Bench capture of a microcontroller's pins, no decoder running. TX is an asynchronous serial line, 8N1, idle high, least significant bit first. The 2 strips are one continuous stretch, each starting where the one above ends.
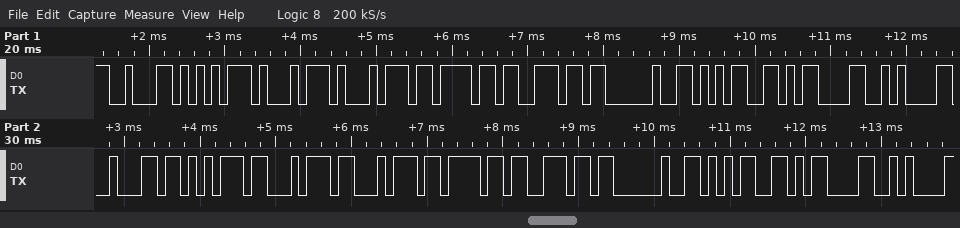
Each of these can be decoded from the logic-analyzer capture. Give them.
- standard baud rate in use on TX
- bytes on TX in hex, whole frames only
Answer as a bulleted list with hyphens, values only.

- 9600 baud
- 0x62 0x75 0x74 0x74 0x6F 0x6E 0x20 0x35 0x0D 0x0A 0x62 0x75 0x74 0x74 0x6F 0x6E 0x20 0x35 0x0D 0x0A
